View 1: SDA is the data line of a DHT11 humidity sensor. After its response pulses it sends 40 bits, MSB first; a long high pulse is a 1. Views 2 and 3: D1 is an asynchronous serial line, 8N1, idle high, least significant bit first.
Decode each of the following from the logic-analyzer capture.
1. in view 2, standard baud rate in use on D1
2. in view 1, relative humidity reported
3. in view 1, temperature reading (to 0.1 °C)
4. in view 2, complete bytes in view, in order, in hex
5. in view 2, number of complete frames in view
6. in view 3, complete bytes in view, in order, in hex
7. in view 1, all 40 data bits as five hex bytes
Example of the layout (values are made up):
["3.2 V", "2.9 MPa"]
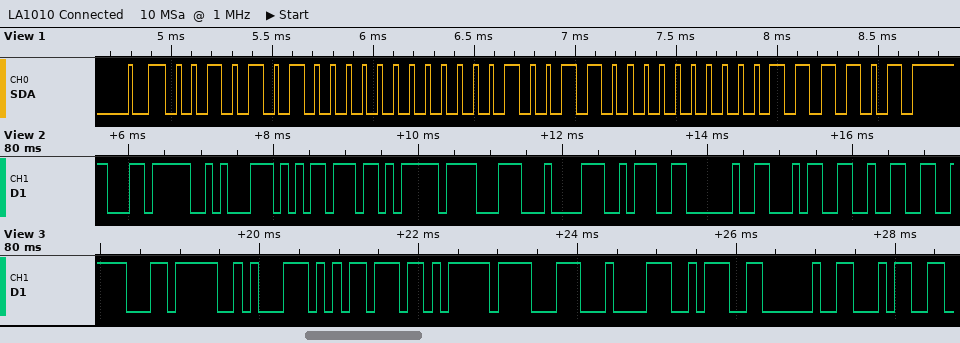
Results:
["9600 baud", "42 %", "19.0 °C", "0xEC 0x8A 0xB5 0xEB 0x8F 0x84 0x3A 0x20 0x34 0x32", "10", "EC 8A B5 EB 8F 84 3A 20 34", "2A 00 13 00 3D"]
